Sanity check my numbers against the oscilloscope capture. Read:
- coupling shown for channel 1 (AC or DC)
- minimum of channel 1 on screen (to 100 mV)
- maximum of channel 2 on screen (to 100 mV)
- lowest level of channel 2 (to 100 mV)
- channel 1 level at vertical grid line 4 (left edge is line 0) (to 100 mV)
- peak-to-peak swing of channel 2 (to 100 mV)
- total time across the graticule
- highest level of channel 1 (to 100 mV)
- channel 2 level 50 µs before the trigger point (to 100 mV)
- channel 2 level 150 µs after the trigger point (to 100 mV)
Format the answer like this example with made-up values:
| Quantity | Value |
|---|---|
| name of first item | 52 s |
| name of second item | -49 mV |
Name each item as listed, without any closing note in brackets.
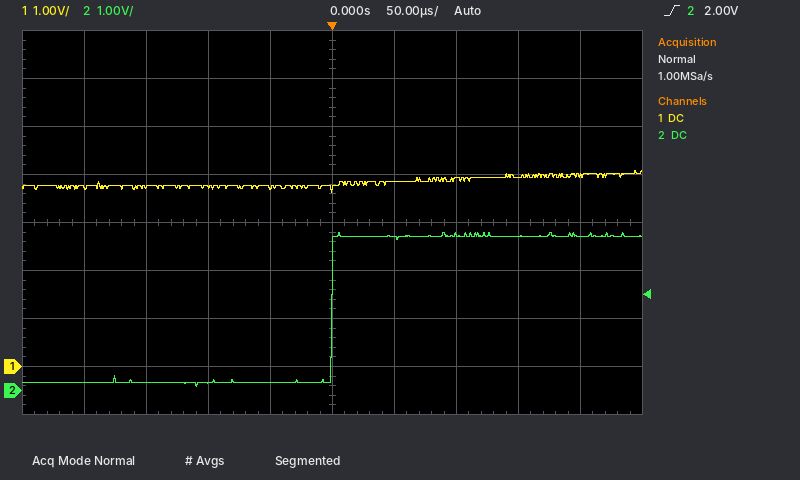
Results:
| Quantity | Value |
|---|---|
| coupling shown for channel 1 | DC |
| minimum of channel 1 on screen | 3.6 V |
| maximum of channel 2 on screen | 3.3 V |
| lowest level of channel 2 | 100 mV |
| channel 1 level at vertical grid line 4 (left edge is line 0) | 3.7 V |
| peak-to-peak swing of channel 2 | 3.2 V |
| total time across the graticule | 500 µs |
| highest level of channel 1 | 4.1 V |
| channel 2 level 50 µs before the trigger point | 200 mV |
| channel 2 level 150 µs after the trigger point | 3.2 V |
